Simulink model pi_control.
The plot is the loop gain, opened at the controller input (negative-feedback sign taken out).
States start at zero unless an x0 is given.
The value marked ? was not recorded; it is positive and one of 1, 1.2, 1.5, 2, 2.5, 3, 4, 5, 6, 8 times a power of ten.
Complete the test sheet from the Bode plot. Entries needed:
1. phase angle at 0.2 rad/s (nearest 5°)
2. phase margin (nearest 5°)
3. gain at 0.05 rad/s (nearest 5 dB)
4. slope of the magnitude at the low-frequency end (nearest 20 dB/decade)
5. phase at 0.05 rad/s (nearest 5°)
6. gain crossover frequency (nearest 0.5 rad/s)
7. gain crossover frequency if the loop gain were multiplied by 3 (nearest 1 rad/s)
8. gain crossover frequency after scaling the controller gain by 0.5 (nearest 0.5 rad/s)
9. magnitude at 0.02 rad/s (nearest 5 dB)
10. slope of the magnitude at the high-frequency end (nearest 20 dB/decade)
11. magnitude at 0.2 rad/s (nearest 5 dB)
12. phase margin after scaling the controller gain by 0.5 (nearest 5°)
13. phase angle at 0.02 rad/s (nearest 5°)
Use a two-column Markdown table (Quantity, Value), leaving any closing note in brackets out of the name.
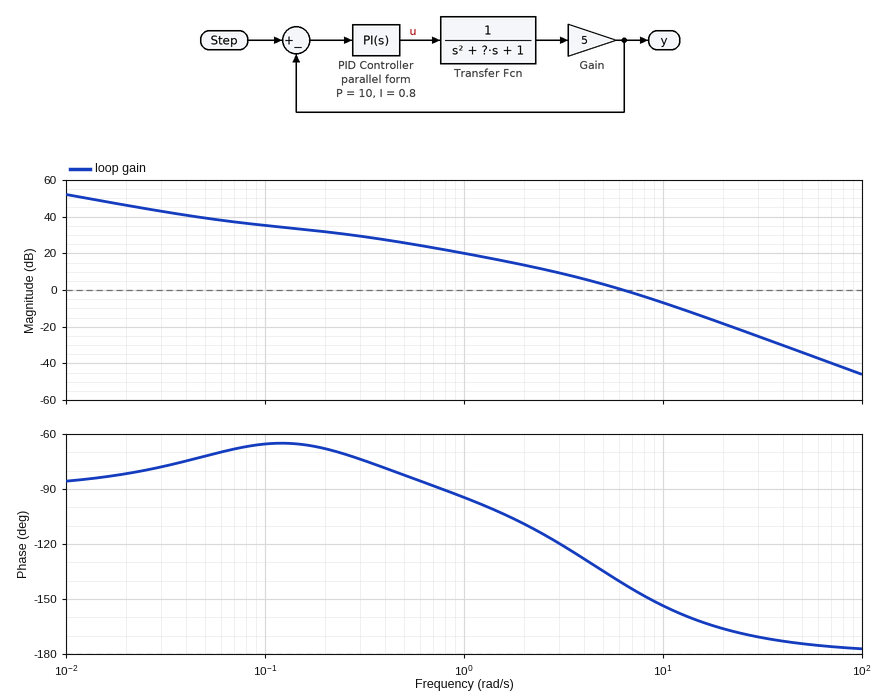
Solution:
| Quantity | Value |
|---|---|
| phase angle at 0.2 rad/s | -70° |
| phase margin | 40° |
| gain at 0.05 rad/s | 40 dB |
| slope of the magnitude at the low-frequency end | -20 dB/decade |
| phase at 0.05 rad/s | -70° |
| gain crossover frequency | 6.5 rad/s |
| gain crossover frequency if the loop gain were multiplied by 3 | 12 rad/s |
| gain crossover frequency after scaling the controller gain by 0.5 | 4.0 rad/s |
| magnitude at 0.02 rad/s | 45 dB |
| slope of the magnitude at the high-frequency end | -40 dB/decade |
| magnitude at 0.2 rad/s | 30 dB |
| phase margin after scaling the controller gain by 0.5 | 50° |
| phase angle at 0.02 rad/s | -80° |
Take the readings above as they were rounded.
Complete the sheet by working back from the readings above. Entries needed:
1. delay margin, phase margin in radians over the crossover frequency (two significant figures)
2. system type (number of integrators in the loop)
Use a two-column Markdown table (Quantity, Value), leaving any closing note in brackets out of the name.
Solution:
| Quantity | Value |
|---|---|
| delay margin, phase margin in radians over the crossover frequency | 0.11 s |
| system type | 1 |
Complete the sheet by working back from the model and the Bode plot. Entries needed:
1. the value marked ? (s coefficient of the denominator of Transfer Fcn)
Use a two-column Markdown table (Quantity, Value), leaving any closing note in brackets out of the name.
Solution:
| Quantity | Value |
|---|---|
| the value marked ? | 5 |
